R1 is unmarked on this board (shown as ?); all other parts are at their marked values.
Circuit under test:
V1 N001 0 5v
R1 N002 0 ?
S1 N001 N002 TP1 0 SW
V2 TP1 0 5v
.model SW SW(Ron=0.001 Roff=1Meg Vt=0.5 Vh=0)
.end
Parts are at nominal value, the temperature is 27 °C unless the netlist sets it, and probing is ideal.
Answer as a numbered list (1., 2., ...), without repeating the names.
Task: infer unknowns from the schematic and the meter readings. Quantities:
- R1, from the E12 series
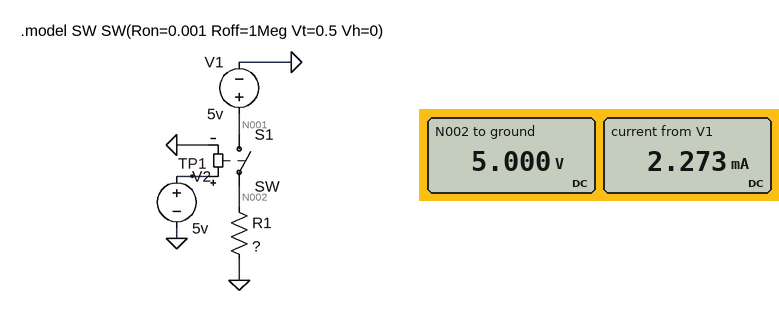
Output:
1. 2.2 kΩ
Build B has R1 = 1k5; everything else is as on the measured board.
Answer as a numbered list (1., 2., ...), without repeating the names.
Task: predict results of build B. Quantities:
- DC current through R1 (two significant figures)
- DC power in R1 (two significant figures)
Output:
1. 3.3 mA
2. 17 mW
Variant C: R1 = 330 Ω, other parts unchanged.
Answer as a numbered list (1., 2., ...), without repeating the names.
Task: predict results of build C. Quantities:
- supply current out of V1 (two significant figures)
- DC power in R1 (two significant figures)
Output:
1. 15 mA
2. 76 mW
